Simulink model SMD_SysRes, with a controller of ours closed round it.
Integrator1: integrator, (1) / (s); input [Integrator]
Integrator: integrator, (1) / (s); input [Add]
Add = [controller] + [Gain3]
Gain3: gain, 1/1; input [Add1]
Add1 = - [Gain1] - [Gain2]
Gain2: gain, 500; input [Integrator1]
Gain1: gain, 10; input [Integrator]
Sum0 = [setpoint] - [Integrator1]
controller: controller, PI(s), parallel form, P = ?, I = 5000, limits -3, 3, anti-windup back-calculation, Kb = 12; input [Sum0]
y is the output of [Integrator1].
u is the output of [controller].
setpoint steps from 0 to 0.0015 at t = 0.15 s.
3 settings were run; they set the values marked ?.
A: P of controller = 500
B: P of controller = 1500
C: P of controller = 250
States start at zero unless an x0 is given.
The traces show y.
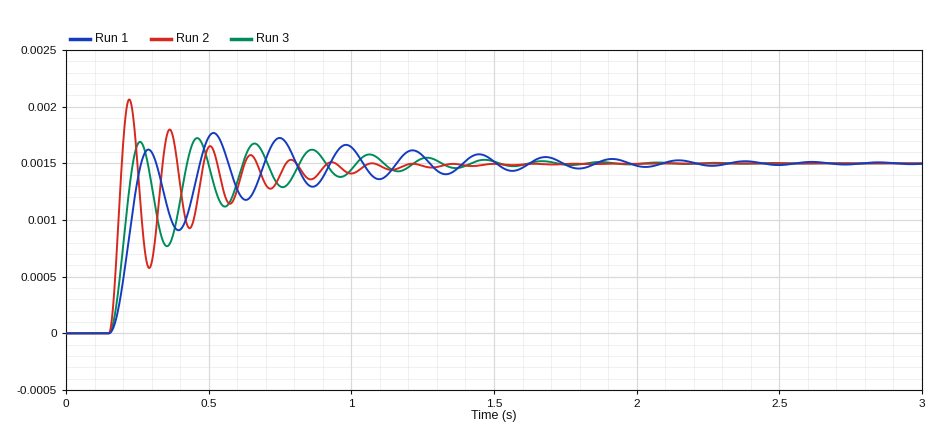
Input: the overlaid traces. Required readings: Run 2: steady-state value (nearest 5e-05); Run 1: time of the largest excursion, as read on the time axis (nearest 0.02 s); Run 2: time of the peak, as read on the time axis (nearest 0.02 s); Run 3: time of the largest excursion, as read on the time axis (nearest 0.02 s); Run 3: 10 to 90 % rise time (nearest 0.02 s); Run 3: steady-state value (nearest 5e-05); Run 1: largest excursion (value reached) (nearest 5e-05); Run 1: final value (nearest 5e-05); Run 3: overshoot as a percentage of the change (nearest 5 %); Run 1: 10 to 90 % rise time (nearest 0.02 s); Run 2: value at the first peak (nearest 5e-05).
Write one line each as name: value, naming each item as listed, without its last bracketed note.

Run 2: steady-state value: 0.00150
Run 1: time of the largest excursion, as read on the time axis: 0.52 s
Run 2: time of the peak, as read on the time axis: 0.22 s
Run 3: time of the largest excursion, as read on the time axis: 0.46 s
Run 3: 10 to 90 % rise time: 0.06 s
Run 3: steady-state value: 0.00150
Run 1: largest excursion (value reached): 0.00175
Run 1: final value: 0.00150
Run 3: overshoot as a percentage of the change: 15 %
Run 1: 10 to 90 % rise time: 0.08 s
Run 2: value at the first peak: 0.00205
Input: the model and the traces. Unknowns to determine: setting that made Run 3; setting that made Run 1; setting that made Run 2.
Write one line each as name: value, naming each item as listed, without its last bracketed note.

setting that made Run 3: A
setting that made Run 1: C
setting that made Run 2: B
